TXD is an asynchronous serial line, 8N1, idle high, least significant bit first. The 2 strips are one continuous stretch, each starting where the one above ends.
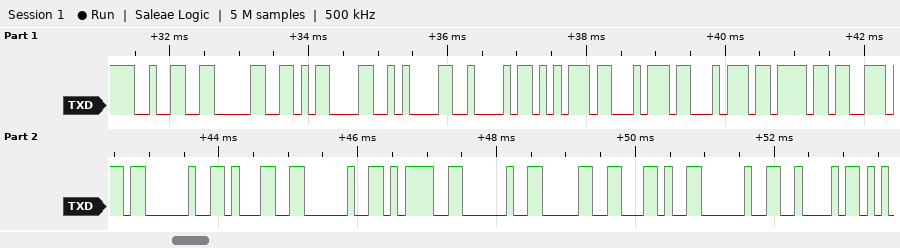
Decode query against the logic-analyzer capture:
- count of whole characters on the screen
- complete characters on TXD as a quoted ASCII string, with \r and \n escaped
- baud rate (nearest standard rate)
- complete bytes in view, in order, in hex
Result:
19
"20\r\nButton 1 = 0, B"
9600 baud
32 30 0D 0A 42 75 74 74 6F 6E 20 31 20 3D 20 30 2C 20 42
